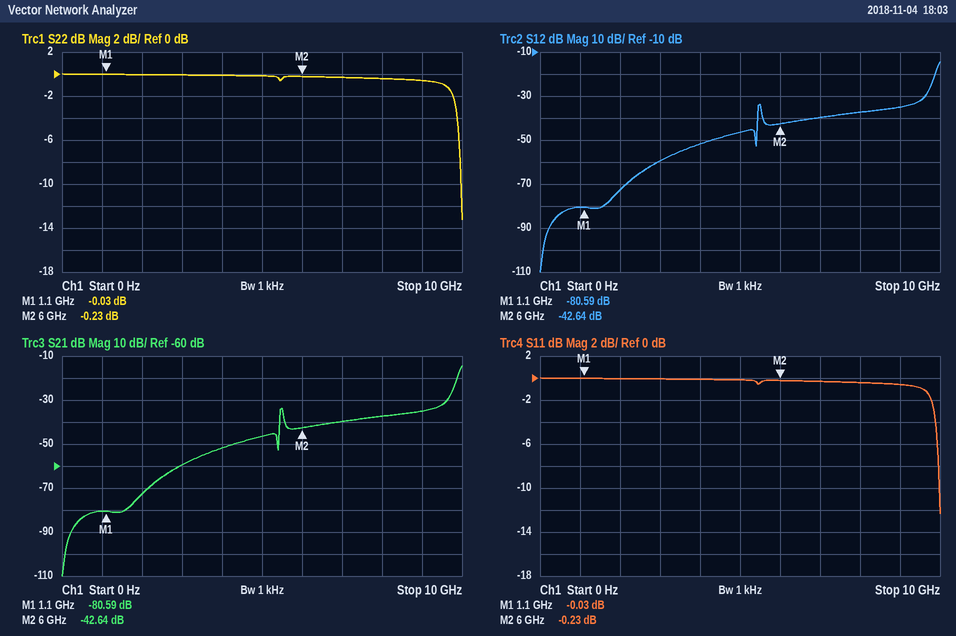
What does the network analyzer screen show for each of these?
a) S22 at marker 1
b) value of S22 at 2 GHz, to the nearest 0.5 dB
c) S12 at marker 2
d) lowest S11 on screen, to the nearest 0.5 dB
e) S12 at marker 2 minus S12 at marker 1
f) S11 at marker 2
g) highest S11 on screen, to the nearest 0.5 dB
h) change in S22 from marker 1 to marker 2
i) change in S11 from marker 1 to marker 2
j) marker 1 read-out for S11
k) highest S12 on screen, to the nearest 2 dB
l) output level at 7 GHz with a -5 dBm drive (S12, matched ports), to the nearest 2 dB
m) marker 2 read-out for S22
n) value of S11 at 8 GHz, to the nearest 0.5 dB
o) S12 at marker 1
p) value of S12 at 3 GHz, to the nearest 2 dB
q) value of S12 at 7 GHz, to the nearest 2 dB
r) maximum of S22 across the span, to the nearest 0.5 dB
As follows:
-0.03 dB
0.0 dB
-42.64 dB
-12.5 dB
37.95 dB
-0.23 dB
0.0 dB
-0.20 dB
-0.20 dB
-0.03 dB
-14 dB
-44 dBm
-0.23 dB
-0.5 dB
-80.59 dB
-60 dB
-40 dB
0.0 dB
